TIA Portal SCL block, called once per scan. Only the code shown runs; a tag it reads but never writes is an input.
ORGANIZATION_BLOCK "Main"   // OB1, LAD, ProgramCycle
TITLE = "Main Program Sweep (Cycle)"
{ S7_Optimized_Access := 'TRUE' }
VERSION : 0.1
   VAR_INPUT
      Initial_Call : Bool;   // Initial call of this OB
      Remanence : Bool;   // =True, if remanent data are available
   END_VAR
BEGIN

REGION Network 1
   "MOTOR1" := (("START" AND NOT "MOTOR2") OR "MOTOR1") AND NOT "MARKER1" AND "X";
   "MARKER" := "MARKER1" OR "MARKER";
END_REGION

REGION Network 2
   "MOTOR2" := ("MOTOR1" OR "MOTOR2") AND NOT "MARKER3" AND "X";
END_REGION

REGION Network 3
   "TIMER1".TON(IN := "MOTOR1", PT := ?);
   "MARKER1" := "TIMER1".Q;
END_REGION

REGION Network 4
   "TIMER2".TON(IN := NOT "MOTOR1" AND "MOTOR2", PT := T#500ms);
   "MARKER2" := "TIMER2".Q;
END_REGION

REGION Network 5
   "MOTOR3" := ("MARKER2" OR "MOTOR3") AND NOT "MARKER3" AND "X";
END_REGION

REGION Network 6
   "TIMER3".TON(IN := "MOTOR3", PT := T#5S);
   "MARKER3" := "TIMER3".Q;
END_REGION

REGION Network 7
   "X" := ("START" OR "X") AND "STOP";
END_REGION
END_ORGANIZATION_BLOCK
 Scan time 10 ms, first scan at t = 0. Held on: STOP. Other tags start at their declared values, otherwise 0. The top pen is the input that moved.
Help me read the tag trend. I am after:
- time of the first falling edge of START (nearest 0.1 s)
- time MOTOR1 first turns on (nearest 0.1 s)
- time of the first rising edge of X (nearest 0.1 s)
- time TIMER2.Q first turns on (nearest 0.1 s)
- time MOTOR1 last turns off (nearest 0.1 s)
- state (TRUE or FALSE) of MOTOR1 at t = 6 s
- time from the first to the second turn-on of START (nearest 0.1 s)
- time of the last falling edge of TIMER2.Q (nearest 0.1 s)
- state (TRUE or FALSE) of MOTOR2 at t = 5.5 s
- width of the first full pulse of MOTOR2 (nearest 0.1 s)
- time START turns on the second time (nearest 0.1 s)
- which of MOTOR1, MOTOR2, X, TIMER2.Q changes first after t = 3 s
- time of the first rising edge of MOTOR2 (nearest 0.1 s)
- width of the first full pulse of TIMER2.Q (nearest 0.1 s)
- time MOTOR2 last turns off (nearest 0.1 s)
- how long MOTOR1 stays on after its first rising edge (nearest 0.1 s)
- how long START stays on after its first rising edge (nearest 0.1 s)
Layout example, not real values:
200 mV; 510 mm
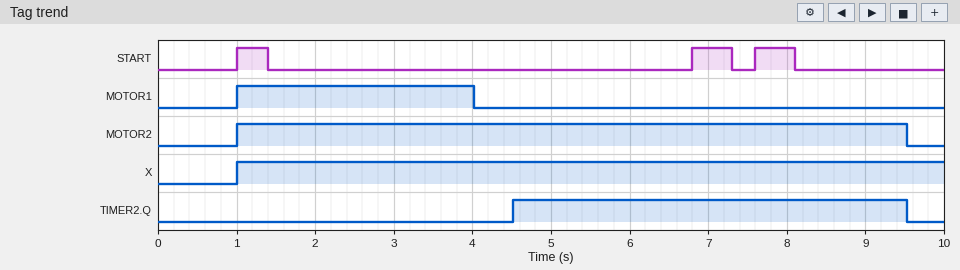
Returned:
1.4 s; 1.0 s; 1.0 s; 4.5 s; 4.0 s; FALSE; 5.8 s; 9.5 s; TRUE; 8.5 s; 6.8 s; MOTOR1; 1.0 s; 5.0 s; 9.5 s; 3.0 s; 0.4 s
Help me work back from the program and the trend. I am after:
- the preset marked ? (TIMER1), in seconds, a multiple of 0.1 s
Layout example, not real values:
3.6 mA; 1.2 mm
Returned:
3.0 s
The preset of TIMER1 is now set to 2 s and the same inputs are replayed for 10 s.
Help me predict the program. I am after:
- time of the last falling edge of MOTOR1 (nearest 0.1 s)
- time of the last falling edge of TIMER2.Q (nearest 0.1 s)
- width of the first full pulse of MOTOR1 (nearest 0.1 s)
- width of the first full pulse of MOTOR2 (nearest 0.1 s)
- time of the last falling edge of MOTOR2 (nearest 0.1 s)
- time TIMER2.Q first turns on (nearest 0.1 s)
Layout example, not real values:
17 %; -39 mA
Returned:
3.0 s; 8.5 s; 2.0 s; 7.5 s; 8.5 s; 3.5 s
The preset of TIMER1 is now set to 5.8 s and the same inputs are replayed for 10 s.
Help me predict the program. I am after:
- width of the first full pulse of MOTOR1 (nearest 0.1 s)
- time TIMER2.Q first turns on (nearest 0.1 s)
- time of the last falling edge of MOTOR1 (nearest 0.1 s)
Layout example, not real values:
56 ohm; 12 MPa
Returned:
5.8 s; 7.3 s; 6.8 s
